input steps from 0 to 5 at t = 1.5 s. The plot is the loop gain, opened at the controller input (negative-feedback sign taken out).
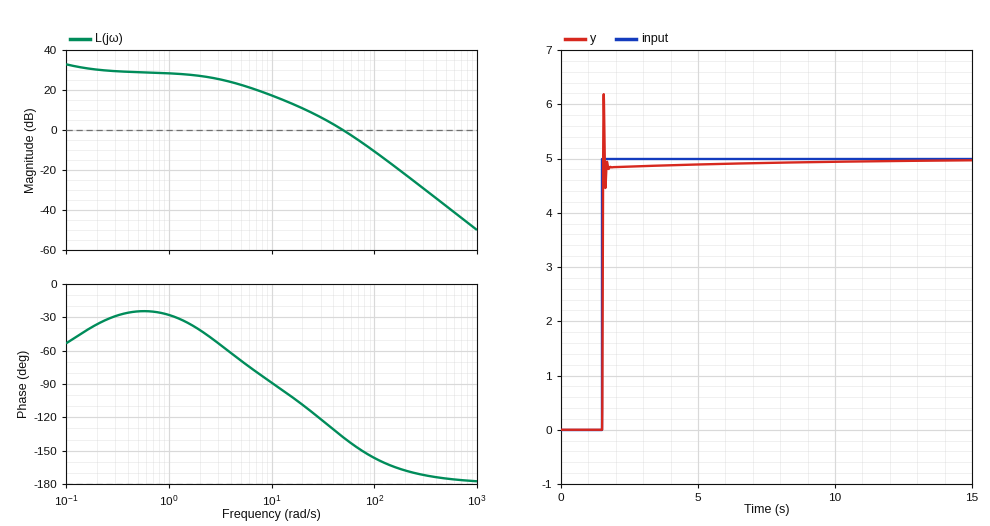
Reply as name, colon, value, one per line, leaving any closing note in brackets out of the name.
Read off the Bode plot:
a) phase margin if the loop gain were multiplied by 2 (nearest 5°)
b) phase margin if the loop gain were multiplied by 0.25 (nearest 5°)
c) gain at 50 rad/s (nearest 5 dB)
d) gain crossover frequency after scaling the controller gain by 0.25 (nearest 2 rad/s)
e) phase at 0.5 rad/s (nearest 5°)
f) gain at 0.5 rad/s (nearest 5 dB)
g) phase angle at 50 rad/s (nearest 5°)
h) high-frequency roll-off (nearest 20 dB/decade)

phase margin if the loop gain were multiplied by 2: 30°
phase margin if the loop gain were multiplied by 0.25: 75°
gain at 50 rad/s: 0 dB
gain crossover frequency after scaling the controller gain by 0.25: 18 rad/s
phase at 0.5 rad/s: -25°
gain at 0.5 rad/s: 30 dB
phase angle at 50 rad/s: -140°
high-frequency roll-off: -40 dB/decade
